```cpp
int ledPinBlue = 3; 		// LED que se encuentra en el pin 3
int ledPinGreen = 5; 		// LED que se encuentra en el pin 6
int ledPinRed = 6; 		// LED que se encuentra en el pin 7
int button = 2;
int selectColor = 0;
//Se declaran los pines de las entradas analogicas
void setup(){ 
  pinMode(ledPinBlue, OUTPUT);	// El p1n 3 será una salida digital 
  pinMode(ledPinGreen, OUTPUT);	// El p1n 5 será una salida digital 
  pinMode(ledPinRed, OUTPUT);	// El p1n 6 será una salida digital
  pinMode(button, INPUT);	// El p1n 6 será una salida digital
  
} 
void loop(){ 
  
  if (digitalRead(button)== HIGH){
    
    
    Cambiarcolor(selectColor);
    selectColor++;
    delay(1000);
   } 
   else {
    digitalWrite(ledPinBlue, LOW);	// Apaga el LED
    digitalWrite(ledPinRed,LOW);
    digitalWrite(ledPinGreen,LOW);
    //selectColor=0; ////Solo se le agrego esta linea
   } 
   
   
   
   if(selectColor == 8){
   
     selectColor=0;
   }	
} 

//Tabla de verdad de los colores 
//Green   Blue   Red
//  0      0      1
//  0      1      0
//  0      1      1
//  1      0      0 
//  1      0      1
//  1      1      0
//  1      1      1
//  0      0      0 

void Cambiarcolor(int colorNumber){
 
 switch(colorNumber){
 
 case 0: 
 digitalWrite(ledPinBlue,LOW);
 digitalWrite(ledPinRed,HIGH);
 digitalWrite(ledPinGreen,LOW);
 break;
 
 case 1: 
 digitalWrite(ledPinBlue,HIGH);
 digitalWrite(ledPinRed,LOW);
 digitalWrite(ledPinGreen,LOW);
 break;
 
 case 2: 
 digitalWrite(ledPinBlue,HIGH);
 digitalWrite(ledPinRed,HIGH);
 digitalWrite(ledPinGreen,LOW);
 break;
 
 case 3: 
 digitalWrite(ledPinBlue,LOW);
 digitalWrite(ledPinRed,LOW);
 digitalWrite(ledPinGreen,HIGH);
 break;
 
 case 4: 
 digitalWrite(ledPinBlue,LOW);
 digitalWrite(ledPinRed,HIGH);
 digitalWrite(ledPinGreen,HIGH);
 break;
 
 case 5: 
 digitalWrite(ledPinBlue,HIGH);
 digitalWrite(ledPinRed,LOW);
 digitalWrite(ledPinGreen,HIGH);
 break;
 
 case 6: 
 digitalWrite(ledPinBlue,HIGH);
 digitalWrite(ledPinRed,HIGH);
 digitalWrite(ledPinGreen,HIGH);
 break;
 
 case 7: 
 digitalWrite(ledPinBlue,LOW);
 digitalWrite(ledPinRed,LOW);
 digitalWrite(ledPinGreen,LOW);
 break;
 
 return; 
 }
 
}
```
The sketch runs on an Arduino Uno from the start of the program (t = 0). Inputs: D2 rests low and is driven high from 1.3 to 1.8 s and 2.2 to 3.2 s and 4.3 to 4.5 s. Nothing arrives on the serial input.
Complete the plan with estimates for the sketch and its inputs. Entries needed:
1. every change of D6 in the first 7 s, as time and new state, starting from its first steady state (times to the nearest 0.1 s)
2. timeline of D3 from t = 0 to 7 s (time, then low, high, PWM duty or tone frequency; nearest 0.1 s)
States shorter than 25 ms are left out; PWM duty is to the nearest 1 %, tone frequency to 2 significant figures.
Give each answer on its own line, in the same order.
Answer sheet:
0 s low; 1.3 s high; 2.3 s low; 4.3 s high; 5.3 s low
0 s low; 2.3 s high; 3.3 s low; 4.3 s high; 5.3 s low
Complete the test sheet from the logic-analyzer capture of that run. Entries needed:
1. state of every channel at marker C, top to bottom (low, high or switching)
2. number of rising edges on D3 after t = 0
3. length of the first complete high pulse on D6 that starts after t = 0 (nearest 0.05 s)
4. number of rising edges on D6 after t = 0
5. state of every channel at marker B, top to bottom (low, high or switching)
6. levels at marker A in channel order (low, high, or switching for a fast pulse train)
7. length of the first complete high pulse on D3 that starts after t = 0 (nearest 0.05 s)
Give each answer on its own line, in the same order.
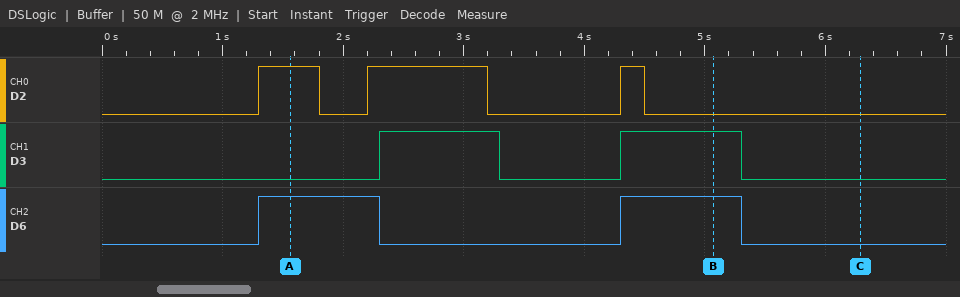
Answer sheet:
D2 low, D3 low, D6 low
2
1.00 s
2
D2 low, D3 high, D6 high
D2 high, D3 low, D6 high
1.00 s
